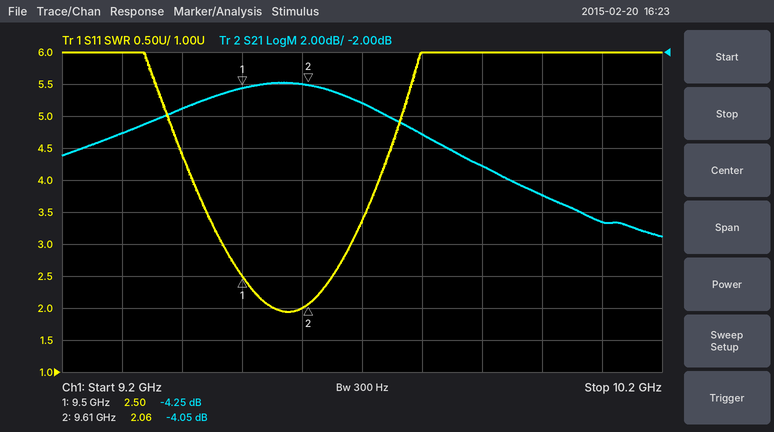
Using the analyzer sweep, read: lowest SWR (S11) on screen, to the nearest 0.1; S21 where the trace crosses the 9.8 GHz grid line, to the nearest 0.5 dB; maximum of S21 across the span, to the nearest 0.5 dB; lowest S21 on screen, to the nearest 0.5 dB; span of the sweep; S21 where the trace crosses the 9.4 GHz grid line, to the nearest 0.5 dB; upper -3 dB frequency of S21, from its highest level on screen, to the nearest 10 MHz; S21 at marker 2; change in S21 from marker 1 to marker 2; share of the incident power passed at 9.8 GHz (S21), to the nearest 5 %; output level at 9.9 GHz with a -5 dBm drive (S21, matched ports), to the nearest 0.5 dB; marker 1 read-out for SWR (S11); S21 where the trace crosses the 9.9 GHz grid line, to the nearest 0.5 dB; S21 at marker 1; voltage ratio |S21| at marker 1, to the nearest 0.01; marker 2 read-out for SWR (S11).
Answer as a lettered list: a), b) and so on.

a) 1.9
b) -7.0 dB
c) -4.0 dB
d) -13.5 dB
e) 1 GHz
f) -5.5 dB
g) 9.79 GHz
h) -4.05 dB
i) 0.20 dB
j) 20 %
k) -14.0 dBm
l) 2.50
m) -9.0 dB
n) -4.25 dB
o) 0.61
p) 2.06
